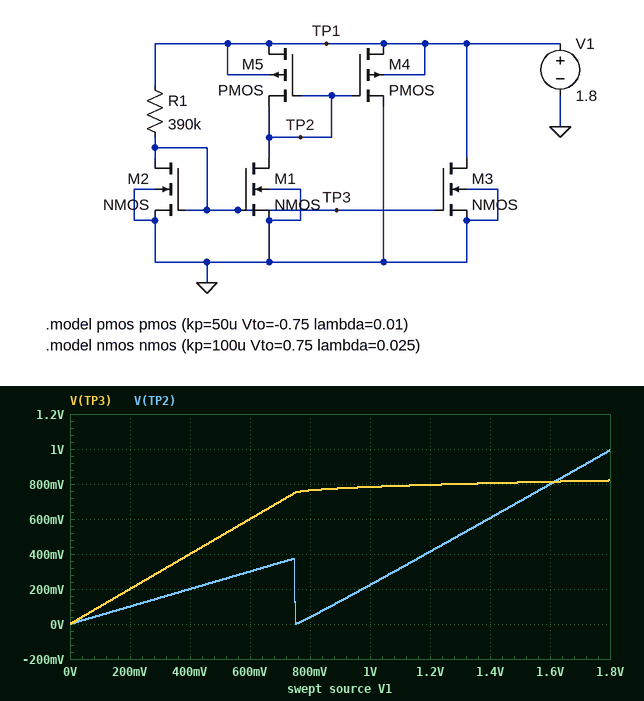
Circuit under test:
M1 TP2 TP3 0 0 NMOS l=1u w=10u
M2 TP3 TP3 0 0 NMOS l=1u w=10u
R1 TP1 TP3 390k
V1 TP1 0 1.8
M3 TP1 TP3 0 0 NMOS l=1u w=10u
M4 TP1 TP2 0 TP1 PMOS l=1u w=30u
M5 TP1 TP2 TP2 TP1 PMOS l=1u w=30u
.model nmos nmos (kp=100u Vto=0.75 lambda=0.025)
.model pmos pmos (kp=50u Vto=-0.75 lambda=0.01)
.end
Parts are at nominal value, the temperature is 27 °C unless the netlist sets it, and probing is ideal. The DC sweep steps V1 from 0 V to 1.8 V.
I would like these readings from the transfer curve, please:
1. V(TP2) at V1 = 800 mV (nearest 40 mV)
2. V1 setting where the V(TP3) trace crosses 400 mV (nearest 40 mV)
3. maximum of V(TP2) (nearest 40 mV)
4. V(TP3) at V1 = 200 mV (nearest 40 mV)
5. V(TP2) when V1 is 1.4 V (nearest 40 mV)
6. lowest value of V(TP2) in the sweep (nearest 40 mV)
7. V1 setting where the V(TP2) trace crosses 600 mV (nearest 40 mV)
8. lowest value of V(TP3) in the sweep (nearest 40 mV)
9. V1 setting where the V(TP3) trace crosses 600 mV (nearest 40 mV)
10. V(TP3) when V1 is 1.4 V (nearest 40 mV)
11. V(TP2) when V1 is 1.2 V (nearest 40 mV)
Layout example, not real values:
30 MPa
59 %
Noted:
40 mV
400 mV
1.00 V
200 mV
600 mV
0 V
1.40 V
0 V
600 mV
800 mV
400 mV
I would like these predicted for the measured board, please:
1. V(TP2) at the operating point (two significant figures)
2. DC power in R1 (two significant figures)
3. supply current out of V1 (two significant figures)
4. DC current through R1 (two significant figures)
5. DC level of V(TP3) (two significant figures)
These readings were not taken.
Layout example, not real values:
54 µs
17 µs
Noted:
990 mV
2.5 µW
10 µA
2.5 µA
820 mV
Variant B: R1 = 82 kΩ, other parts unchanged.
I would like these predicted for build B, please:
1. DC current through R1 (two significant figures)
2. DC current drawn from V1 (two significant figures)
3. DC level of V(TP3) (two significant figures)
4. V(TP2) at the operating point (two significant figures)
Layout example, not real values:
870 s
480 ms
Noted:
11 µA
44 µA
900 mV
930 mV
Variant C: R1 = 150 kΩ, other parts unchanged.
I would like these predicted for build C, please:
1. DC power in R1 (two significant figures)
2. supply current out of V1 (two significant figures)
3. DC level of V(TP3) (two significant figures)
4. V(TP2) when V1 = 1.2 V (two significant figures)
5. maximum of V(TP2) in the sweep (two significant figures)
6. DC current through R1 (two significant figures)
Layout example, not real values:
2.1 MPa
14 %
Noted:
5.9 µW
25 µA
860 mV
390 mV
960 mV
6.3 µA
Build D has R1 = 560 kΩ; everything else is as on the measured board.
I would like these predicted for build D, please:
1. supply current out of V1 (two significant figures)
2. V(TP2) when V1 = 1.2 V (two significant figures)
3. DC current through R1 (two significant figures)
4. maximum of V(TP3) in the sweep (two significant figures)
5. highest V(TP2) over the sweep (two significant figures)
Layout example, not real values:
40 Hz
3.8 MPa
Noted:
7.2 µA
420 mV
1.8 µA
810 mV
1.0 V
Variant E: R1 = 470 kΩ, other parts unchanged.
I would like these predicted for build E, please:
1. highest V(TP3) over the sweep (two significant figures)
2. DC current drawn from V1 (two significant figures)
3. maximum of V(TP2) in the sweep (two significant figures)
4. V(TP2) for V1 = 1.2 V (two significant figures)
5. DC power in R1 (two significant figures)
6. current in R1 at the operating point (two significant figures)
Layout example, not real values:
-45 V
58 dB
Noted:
810 mV
8.5 µA
1.0 V
420 mV
2.1 µW
2.1 µA
